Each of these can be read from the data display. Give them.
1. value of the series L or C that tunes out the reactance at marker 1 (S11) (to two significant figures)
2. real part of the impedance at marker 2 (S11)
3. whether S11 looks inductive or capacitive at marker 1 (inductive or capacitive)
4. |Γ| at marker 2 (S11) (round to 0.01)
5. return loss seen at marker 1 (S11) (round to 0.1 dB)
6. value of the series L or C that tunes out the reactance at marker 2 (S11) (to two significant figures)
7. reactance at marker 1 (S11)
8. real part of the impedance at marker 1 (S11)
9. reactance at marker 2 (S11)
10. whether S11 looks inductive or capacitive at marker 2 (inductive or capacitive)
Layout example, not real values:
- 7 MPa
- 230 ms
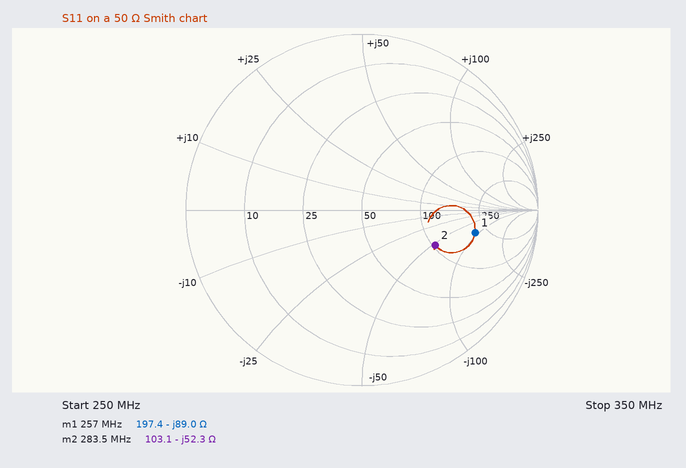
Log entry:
- 55 nH
- 103.1 Ω
- capacitive
- 0.46
- 3.7 dB
- 29 nH
- -89.0 Ω
- 197.4 Ω
- -52.3 Ω
- capacitive
